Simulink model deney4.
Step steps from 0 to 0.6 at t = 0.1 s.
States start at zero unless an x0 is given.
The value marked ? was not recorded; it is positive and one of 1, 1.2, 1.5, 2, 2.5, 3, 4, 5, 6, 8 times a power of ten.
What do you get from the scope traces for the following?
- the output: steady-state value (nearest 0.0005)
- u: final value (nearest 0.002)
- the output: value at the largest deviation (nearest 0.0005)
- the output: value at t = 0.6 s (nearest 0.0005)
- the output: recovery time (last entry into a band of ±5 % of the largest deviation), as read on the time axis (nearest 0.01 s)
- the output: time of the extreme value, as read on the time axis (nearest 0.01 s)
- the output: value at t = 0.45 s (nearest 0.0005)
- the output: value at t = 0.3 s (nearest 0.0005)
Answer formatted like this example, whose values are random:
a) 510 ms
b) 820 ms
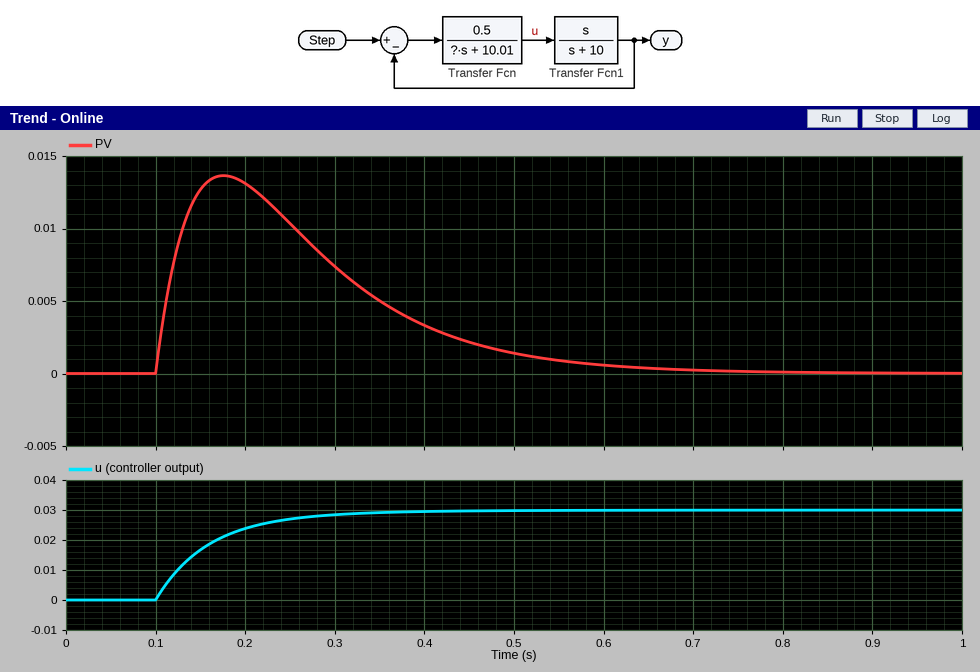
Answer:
a) 0.0000
b) 0.030
c) 0.0135
d) 0.0005
e) 0.58 s
f) 0.18 s
g) 0.0020
h) 0.0075
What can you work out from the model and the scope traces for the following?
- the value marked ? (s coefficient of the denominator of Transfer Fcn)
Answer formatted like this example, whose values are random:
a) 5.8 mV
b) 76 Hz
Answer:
a) 0.6
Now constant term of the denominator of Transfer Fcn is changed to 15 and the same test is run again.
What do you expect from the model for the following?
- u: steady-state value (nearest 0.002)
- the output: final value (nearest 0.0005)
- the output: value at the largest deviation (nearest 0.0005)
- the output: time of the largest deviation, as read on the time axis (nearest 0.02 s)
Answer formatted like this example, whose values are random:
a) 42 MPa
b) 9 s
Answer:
a) 0.020
b) 0.0000
c) 0.0105
d) 0.16 s
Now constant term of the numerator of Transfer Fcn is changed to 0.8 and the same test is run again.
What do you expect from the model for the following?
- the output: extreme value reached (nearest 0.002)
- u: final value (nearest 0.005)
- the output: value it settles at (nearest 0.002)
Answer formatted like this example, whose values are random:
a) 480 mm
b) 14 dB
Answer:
a) 0.022
b) 0.050
c) 0.000
